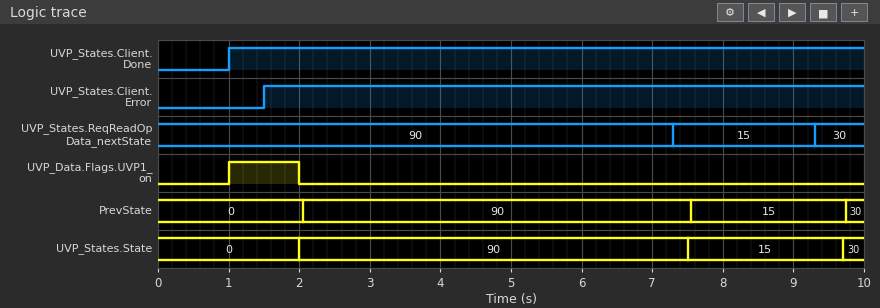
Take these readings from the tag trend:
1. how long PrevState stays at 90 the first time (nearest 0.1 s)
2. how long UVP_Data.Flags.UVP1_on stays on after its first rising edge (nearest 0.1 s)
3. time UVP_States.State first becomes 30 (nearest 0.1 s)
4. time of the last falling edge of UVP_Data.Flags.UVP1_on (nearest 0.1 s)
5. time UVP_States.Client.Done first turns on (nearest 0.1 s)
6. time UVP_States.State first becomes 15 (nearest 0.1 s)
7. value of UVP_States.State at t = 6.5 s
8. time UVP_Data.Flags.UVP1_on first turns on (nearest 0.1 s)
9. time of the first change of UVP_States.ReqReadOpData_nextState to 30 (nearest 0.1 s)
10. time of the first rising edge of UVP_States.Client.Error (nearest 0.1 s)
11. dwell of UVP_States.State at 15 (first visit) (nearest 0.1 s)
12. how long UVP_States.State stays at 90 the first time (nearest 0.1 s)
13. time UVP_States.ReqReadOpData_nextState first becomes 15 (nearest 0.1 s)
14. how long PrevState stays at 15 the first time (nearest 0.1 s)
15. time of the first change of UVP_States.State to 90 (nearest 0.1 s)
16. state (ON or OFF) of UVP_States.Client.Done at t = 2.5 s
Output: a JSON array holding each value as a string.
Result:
["5.5 s", "1.0 s", "9.7 s", "2.0 s", "1.0 s", "7.5 s", "90", "1.0 s", "9.3 s", "1.5 s", "2.2 s", "5.5 s", "7.3 s", "2.2 s", "2.0 s", "ON"]
